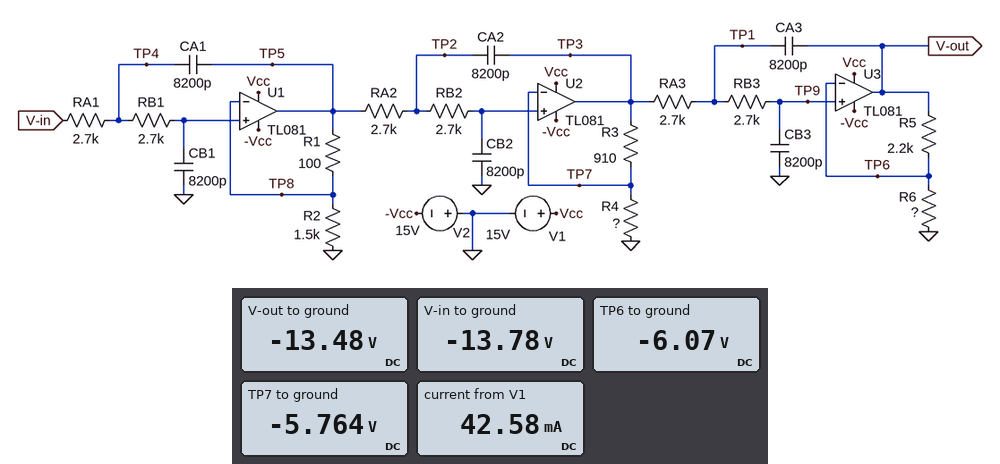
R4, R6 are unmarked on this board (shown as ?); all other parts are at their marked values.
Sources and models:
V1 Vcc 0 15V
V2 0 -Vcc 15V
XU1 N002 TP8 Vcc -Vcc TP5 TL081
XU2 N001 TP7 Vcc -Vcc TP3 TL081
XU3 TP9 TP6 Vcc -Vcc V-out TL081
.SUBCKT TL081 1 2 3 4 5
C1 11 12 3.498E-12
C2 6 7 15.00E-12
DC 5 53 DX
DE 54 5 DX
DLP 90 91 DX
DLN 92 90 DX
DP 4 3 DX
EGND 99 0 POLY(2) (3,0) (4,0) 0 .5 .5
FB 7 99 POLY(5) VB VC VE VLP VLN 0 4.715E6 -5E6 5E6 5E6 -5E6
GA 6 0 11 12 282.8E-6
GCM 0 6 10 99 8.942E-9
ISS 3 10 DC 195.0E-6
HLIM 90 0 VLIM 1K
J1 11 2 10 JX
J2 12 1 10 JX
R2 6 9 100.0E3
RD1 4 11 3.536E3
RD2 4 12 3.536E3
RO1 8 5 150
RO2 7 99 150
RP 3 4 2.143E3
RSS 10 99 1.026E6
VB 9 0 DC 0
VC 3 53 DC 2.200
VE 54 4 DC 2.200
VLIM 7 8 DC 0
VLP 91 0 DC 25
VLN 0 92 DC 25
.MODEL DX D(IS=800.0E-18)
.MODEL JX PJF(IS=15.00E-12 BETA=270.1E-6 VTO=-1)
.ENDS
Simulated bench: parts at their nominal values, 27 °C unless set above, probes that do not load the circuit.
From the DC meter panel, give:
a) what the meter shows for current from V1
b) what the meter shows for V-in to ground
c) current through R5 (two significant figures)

42.58 mA
-13.78 V
3.4 mA
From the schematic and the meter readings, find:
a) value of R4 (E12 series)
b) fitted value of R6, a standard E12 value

680 Ω
1.8 kΩ
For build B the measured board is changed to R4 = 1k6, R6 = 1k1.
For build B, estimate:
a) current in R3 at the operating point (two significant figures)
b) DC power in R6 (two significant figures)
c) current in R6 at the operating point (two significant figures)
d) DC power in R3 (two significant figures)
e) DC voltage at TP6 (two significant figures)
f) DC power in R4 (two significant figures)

5.4 mA
18 mW
4.1 mA
26 mW
-4.5 V
46 mW
